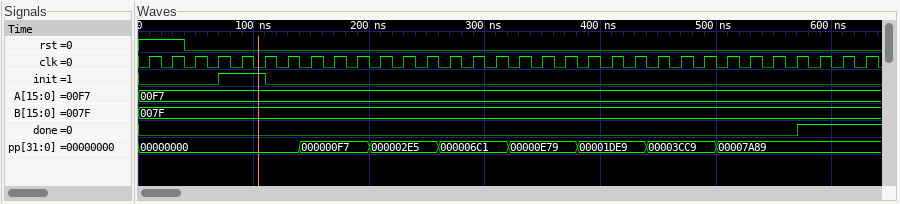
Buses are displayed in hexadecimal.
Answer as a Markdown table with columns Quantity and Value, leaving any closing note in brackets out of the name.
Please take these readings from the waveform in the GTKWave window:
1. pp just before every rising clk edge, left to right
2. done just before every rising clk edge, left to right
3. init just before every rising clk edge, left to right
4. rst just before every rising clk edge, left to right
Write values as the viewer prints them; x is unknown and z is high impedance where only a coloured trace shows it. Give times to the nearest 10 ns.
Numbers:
| Quantity | Value |
|---|---|
| pp just before every rising clk edge, left to right | 00000000, 00000000, 00000000, 00000000, 00000000, 00000000, 00000000, 000000F7, 000000F7, 000000F7, 000002E5, 000002E5, 000002E5, 000006C1, 000006C1, 000006C1, 00000E79, 00000E79, 00000E79, 00001DE9, 00001DE9, 00001DE9, 00003CC9, 00003CC9, 00003CC9, 00007A89, 00007A89, 00007A89, 00007A89, 00007A89, 00007A89, 00007A89 |
| done just before every rising clk edge, left to right | 0 0 0 0 0 0 0 0 0 0 0 0 0 0 0 0 0 0 0 0 0 0 0 0 0 0 0 0 0 1 1 1 |
| init just before every rising clk edge, left to right | 0 0 0 0 1 1 0 0 0 0 0 0 0 0 0 0 0 0 0 0 0 0 0 0 0 0 0 0 0 0 0 0 |
| rst just before every rising clk edge, left to right | 1 1 0 0 0 0 0 0 0 0 0 0 0 0 0 0 0 0 0 0 0 0 0 0 0 0 0 0 0 0 0 0 |
